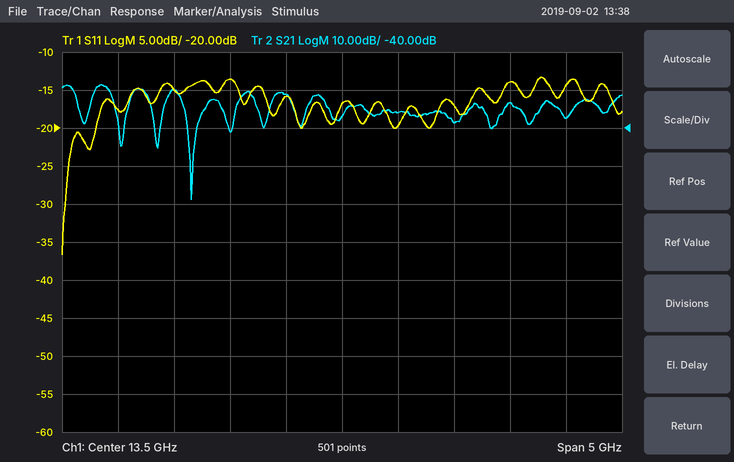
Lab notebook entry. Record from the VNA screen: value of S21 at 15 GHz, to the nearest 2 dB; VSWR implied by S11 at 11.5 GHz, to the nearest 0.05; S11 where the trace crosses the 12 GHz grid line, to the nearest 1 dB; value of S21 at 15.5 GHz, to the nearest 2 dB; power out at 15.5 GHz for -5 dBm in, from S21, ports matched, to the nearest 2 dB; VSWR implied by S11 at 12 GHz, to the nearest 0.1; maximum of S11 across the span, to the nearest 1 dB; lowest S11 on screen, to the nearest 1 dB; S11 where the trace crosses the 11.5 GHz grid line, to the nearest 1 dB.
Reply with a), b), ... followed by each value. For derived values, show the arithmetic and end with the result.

a) -34 dB
b) |Γ| = 10^(-18/20) = 0.1259; VSWR = (1 + 0.1259)/(1 − 0.1259) ≈ 1.29, so 1.30 to the nearest 0.05
c) -15 dB
d) -38 dB
e) -5 dBm + (-38 dB) = -42 dBm
f) |Γ| = 10^(-15/20) = 0.1778; VSWR = (1 + 0.1778)/(1 − 0.1778) ≈ 1.4
g) -13 dB
h) -37 dB
i) -18 dB
